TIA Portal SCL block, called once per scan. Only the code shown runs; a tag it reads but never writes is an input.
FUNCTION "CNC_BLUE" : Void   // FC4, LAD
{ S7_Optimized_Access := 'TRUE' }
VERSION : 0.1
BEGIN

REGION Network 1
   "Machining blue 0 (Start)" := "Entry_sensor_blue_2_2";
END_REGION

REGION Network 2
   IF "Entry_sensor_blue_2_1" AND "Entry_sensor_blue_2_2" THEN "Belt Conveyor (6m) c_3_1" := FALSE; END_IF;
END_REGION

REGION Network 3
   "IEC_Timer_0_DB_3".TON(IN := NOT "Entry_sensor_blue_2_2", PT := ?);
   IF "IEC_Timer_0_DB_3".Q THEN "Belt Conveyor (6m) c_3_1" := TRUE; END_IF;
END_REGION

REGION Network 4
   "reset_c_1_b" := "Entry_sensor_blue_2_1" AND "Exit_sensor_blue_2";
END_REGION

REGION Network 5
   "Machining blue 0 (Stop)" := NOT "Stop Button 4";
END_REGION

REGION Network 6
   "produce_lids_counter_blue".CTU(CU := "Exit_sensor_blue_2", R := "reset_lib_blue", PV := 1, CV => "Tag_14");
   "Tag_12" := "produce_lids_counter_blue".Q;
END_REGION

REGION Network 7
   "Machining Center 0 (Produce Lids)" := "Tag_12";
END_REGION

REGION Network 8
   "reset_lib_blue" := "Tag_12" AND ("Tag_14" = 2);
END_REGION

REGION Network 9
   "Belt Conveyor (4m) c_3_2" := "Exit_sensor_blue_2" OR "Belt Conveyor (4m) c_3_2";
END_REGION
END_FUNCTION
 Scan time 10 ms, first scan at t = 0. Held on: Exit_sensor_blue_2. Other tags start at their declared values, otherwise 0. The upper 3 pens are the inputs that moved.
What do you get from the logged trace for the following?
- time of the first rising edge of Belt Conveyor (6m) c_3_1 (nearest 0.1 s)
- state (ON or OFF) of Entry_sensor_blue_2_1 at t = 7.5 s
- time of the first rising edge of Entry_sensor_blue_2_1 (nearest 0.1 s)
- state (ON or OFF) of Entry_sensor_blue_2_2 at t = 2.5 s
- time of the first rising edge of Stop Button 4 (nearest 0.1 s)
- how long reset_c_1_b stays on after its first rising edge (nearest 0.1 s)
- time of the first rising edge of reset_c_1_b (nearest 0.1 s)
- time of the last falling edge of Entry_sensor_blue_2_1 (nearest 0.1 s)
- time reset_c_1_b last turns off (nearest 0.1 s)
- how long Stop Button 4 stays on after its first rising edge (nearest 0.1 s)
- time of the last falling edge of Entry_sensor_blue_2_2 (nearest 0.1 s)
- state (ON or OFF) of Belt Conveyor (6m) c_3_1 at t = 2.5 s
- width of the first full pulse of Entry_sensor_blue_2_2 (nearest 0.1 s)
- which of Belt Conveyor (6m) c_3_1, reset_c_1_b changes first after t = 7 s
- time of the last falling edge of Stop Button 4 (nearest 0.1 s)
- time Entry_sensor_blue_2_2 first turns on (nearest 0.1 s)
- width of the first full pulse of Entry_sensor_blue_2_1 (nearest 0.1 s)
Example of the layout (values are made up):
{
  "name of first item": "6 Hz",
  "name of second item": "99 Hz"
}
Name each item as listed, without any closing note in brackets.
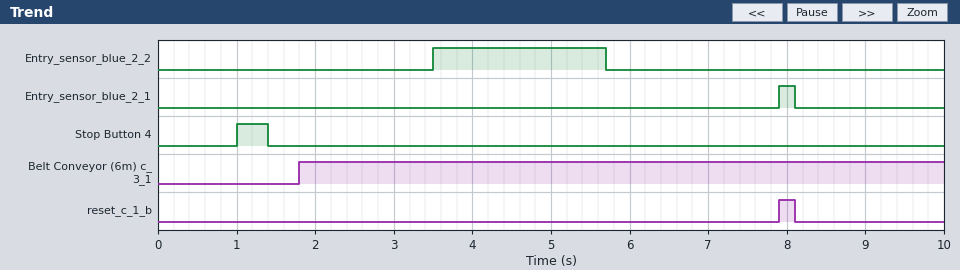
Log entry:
{
  "time of the first rising edge of Belt Conveyor (6m) c_3_1": "1.8 s",
  "state (ON or OFF) of Entry_sensor_blue_2_1 at t = 7.5 s": "OFF",
  "time of the first rising edge of Entry_sensor_blue_2_1": "7.9 s",
  "state (ON or OFF) of Entry_sensor_blue_2_2 at t = 2.5 s": "OFF",
  "time of the first rising edge of Stop Button 4": "1.0 s",
  "how long reset_c_1_b stays on after its first rising edge": "0.2 s",
  "time of the first rising edge of reset_c_1_b": "7.9 s",
  "time of the last falling edge of Entry_sensor_blue_2_1": "8.1 s",
  "time reset_c_1_b last turns off": "8.1 s",
  "how long Stop Button 4 stays on after its first rising edge": "0.4 s",
  "time of the last falling edge of Entry_sensor_blue_2_2": "5.7 s",
  "state (ON or OFF) of Belt Conveyor (6m) c_3_1 at t = 2.5 s": "ON",
  "width of the first full pulse of Entry_sensor_blue_2_2": "2.2 s",
  "which of Belt Conveyor (6m) c_3_1, reset_c_1_b changes first after t = 7 s": "reset_c_1_b",
  "time of the last falling edge of Stop Button 4": "1.4 s",
  "time Entry_sensor_blue_2_2 first turns on": "3.5 s",
  "width of the first full pulse of Entry_sensor_blue_2_1": "0.2 s"
}
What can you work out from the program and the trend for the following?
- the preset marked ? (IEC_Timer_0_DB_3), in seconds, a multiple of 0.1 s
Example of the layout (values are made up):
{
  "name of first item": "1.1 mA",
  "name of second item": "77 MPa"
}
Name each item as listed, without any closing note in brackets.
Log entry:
{
  "the preset marked ? (IEC_Timer_0_DB_3), in seconds, a multiple of 0.1 s": "1.8 s"
}
